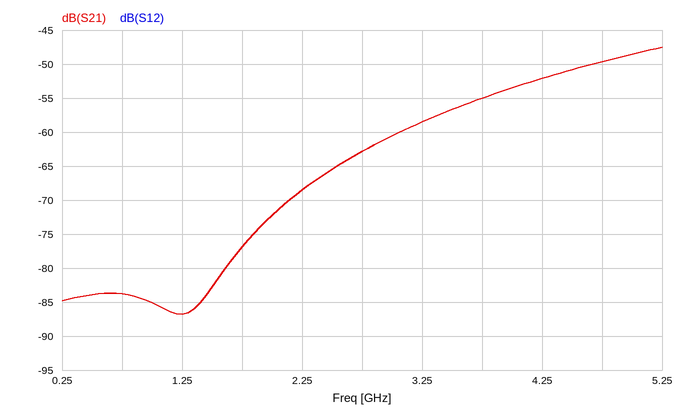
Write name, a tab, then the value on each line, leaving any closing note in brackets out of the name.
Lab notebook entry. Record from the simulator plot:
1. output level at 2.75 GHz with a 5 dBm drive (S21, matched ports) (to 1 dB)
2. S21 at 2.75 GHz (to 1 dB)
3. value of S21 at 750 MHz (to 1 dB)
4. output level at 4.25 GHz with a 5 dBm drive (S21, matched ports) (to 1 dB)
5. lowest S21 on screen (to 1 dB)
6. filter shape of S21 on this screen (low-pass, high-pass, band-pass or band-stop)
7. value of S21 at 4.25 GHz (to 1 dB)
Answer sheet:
output level at 2.75 GHz with a 5 dBm drive (S21, matched ports)	-58 dBm
S21 at 2.75 GHz	-63 dB
value of S21 at 750 MHz	-84 dB
output level at 4.25 GHz with a 5 dBm drive (S21, matched ports)	-47 dBm
lowest S21 on screen	-87 dB
filter shape of S21 on this screen	high-pass
value of S21 at 4.25 GHz	-52 dB
